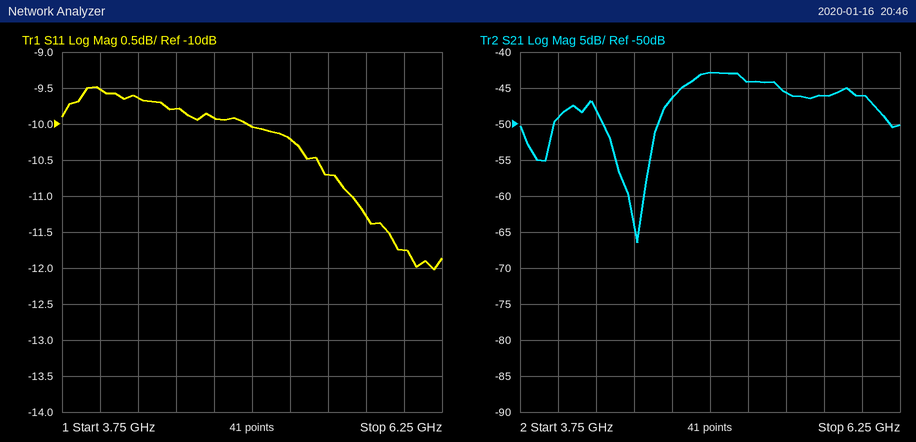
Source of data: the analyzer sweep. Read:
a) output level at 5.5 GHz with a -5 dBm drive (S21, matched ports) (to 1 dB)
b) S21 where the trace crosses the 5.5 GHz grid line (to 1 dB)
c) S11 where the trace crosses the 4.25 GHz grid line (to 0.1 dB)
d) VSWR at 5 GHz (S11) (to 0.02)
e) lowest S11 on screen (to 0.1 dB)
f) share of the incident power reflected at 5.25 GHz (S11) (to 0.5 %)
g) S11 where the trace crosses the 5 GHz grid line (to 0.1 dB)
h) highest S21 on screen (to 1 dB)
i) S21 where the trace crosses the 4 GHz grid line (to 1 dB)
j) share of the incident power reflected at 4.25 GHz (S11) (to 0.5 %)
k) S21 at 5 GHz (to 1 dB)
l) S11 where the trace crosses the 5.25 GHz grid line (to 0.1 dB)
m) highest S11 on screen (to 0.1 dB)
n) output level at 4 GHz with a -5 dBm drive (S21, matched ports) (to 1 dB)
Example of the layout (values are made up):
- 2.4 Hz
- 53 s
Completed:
- -51 dBm
- -46 dB
- -9.6 dB
- 1.92
- -12.0 dB
- 9.5 %
- -10.0 dB
- -43 dB
- -49 dB
- 11.0 %
- -43 dB
- -10.2 dB
- -9.5 dB
- -54 dBm
